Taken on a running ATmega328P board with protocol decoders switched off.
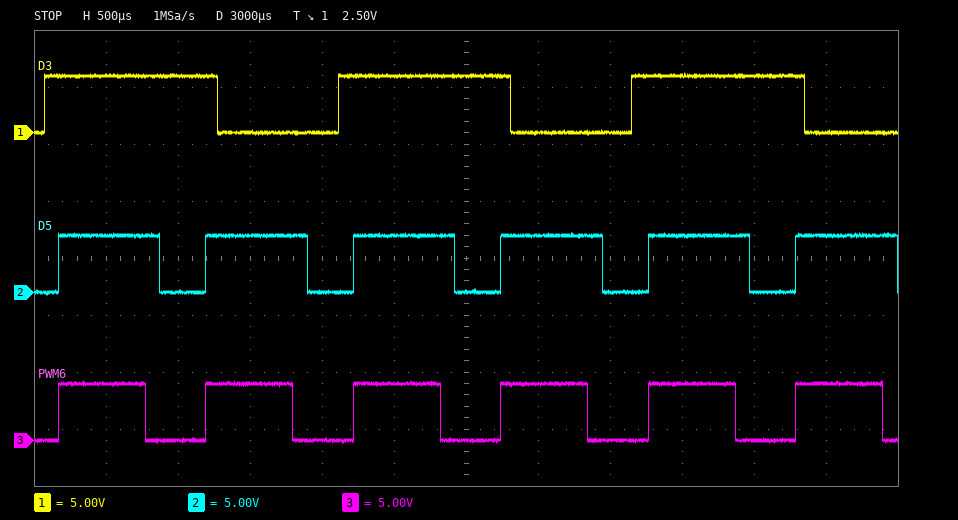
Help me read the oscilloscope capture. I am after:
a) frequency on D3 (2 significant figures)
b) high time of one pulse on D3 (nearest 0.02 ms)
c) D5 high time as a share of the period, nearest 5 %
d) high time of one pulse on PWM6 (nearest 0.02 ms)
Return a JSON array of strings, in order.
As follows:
["490 Hz", "1.20 ms", "70 %", "0.60 ms"]
